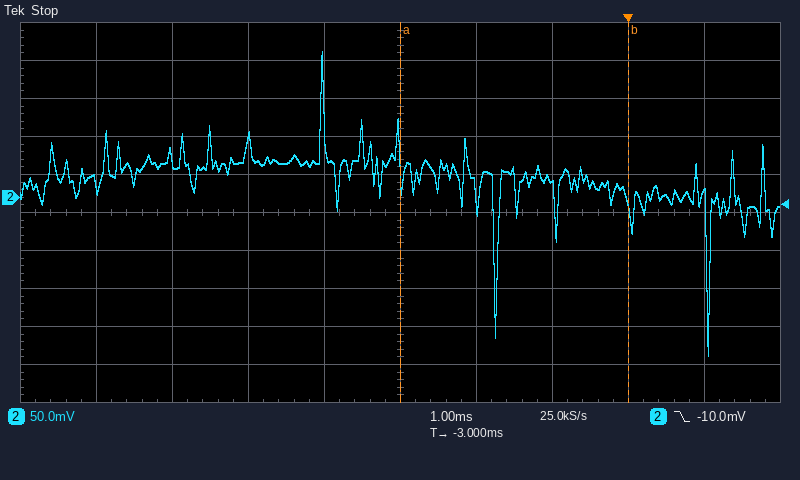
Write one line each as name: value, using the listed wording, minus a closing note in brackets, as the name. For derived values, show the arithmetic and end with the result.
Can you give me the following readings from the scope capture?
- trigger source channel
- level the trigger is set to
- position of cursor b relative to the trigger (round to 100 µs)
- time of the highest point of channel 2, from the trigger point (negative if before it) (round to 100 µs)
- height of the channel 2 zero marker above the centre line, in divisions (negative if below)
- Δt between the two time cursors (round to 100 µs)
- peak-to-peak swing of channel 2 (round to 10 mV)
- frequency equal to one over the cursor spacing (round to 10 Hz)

trigger source channel: channel 2
level the trigger is set to: -10.0 mV
position of cursor b relative to the trigger: 0.0 ms
time of the highest point of channel 2, from the trigger point (negative if before it): -4.0 ms
height of the channel 2 zero marker above the centre line, in divisions: +0.4 div
Δt between the two time cursors: 3.0 ms
peak-to-peak swing of channel 2: 400 mV
frequency equal to one over the cursor spacing: 1 / 3.0 ms ≈ 330 Hz
